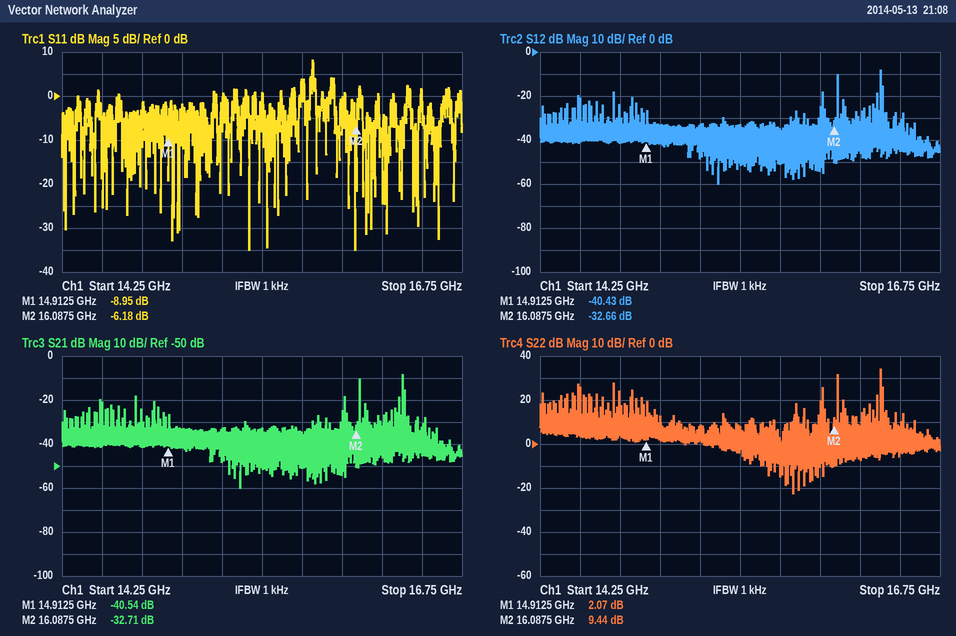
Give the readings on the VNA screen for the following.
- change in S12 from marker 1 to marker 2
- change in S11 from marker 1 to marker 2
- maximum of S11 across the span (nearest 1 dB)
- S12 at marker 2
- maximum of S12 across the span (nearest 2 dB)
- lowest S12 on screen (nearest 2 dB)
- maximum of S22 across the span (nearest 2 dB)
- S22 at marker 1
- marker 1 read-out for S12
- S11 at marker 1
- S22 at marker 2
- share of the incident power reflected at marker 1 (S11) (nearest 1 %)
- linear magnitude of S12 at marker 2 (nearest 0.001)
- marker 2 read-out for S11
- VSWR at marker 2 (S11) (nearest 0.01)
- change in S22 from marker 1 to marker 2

7.77 dB
2.77 dB
8 dB
-32.66 dB
-8 dB
-60 dB
34 dB
2.07 dB
-40.43 dB
-8.95 dB
9.44 dB
13 %
0.023
-6.18 dB
2.93
7.37 dB
